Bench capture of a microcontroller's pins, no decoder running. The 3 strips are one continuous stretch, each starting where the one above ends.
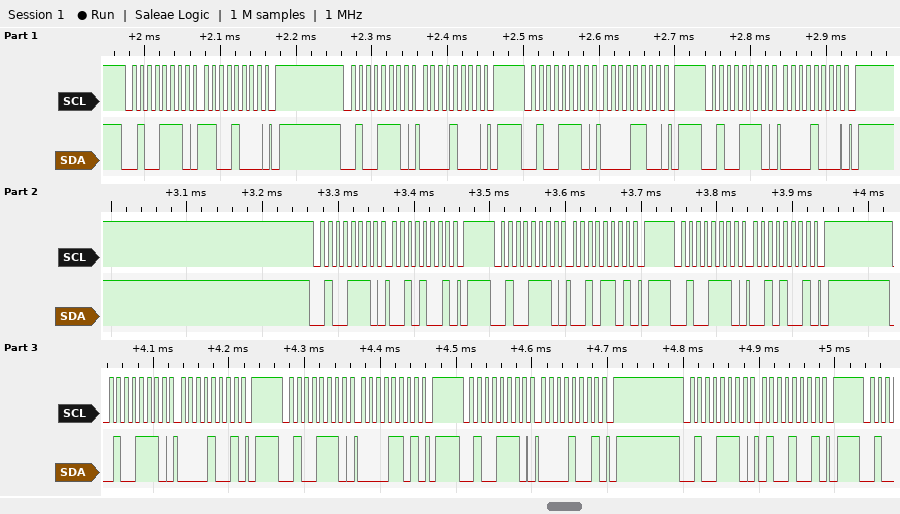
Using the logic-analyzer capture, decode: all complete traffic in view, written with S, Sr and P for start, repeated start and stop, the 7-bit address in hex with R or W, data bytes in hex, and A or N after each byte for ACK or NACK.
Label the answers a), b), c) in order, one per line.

a) S 27W A C8 A P S 27W A 08 A P S 27W A 0C A P S 27W A 08 A P S 27W A 29 A P S 27W A 2D A P S 27W A 29 A P S 27W A 09 A P S 27W A 0D A P S 27W A 09 A P S 27W A 49 A P
